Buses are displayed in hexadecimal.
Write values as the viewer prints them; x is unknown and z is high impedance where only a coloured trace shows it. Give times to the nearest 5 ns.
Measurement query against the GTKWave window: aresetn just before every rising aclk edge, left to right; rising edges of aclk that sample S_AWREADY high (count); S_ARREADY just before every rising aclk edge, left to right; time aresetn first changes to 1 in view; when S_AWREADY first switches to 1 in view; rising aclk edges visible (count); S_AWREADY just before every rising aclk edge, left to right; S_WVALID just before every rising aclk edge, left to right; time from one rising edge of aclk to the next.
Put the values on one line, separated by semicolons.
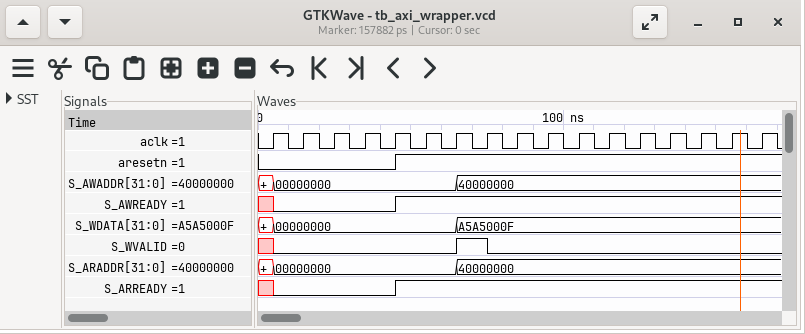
0 0 0 0 0 1 1 1 1 1 1 1 1 1 1 1 1; 12; x 0 0 0 0 1 1 1 1 1 1 1 1 1 1 1 1; 45 ns; 45 ns; 17; x 0 0 0 0 1 1 1 1 1 1 1 1 1 1 1 1; x 0 0 0 0 0 0 1 0 0 0 0 0 0 0 0 0; 10 ns
